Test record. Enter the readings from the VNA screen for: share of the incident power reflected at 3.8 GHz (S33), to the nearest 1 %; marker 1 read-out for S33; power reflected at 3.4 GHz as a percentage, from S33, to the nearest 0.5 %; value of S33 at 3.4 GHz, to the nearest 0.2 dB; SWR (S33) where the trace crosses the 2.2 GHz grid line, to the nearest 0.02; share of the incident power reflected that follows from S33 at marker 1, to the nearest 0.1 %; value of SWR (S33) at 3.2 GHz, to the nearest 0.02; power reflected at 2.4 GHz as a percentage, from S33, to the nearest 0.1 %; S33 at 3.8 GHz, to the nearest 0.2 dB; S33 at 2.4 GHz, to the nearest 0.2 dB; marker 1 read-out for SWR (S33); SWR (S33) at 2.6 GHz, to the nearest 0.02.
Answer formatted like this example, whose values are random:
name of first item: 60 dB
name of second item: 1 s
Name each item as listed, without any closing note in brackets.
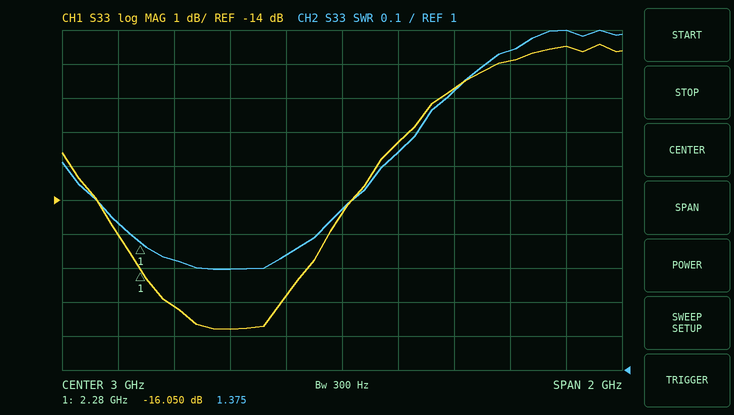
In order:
share of the incident power reflected at 3.8 GHz (S33), to the nearest 1 %: 11 %
marker 1 read-out for S33: -16.050 dB
power reflected at 3.4 GHz as a percentage, from S33, to the nearest 0.5 %: 8.5 %
value of S33 at 3.4 GHz, to the nearest 0.2 dB: -10.8 dB
SWR (S33) where the trace crosses the 2.2 GHz grid line, to the nearest 0.02: 1.44
share of the incident power reflected that follows from S33 at marker 1, to the nearest 0.1 %: 2.5 %
value of SWR (S33) at 3.2 GHz, to the nearest 0.02: 1.64
power reflected at 2.4 GHz as a percentage, from S33, to the nearest 0.1 %: 1.9 %
S33 at 3.8 GHz, to the nearest 0.2 dB: -9.4 dB
S33 at 2.4 GHz, to the nearest 0.2 dB: -17.2 dB
marker 1 read-out for SWR: 1.375
SWR (S33) at 2.6 GHz, to the nearest 0.02: 1.30
